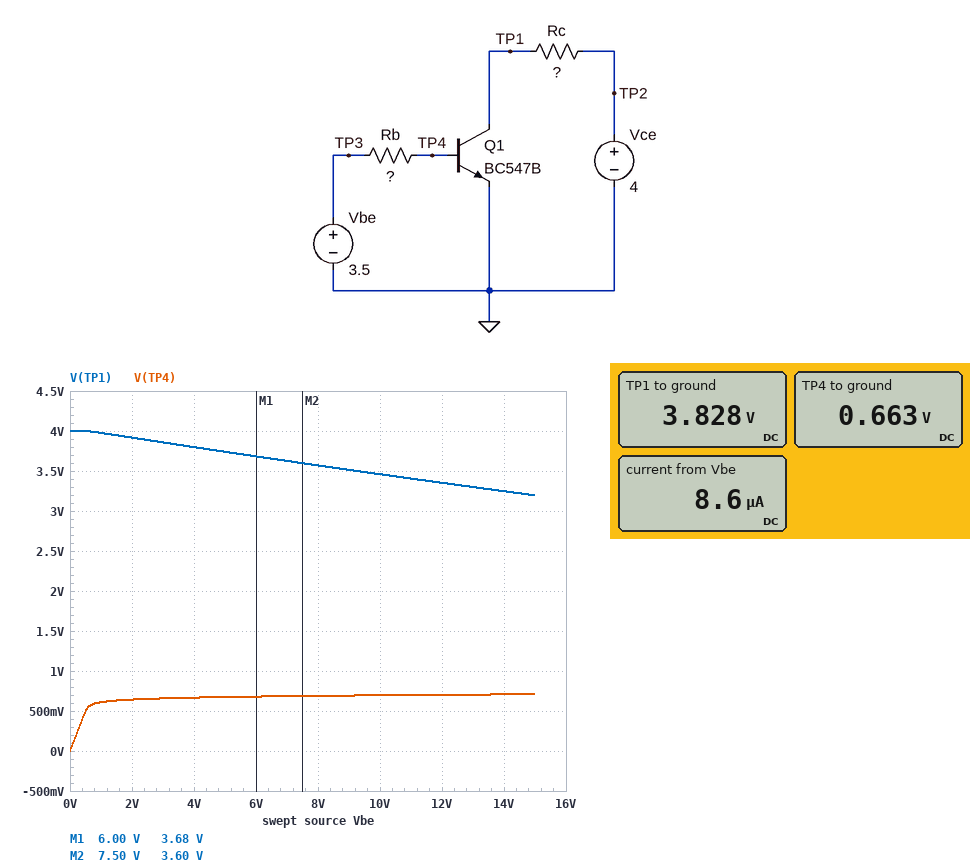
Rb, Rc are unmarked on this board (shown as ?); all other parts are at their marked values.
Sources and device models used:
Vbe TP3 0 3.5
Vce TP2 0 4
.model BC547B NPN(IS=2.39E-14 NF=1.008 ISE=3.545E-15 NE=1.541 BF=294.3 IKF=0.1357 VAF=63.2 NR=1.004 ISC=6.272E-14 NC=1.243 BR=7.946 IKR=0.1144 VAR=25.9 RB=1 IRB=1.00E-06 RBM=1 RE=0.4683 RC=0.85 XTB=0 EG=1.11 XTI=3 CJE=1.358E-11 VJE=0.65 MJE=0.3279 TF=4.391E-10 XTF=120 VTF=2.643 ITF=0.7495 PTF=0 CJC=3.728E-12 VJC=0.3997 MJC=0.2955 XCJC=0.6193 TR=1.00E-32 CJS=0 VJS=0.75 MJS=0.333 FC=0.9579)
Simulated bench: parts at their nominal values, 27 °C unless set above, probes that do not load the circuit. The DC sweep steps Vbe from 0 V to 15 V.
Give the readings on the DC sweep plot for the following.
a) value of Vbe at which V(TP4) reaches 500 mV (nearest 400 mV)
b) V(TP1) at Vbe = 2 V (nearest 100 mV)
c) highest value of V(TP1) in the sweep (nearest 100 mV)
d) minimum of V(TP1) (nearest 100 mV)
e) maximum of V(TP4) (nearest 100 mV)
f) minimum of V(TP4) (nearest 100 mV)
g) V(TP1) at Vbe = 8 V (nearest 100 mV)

400 mV
3.9 V
4.0 V
3.2 V
700 mV
0 V
3.6 V
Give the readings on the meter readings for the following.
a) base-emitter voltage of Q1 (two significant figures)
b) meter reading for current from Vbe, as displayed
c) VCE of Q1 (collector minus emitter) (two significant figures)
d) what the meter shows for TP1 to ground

660 mV
8.6 µA
3.8 V
3.828 V
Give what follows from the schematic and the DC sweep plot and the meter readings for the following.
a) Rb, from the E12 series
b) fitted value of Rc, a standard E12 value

330 kΩ
68 Ω
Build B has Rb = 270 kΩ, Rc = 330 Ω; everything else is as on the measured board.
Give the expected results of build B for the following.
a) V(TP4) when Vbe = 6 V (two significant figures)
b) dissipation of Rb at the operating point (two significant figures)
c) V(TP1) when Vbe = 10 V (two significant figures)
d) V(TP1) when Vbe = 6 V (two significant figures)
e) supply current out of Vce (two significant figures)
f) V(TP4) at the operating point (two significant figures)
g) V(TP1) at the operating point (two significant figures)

690 mV
30 µW
960 mV
2.2 V
3.0 mA
670 mV
3.0 V
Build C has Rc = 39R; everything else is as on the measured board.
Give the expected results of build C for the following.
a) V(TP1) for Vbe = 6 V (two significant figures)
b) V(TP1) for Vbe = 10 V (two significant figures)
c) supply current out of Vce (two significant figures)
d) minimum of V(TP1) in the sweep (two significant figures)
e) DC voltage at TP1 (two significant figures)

3.8 V
3.7 V
2.5 mA
3.5 V
3.9 V
